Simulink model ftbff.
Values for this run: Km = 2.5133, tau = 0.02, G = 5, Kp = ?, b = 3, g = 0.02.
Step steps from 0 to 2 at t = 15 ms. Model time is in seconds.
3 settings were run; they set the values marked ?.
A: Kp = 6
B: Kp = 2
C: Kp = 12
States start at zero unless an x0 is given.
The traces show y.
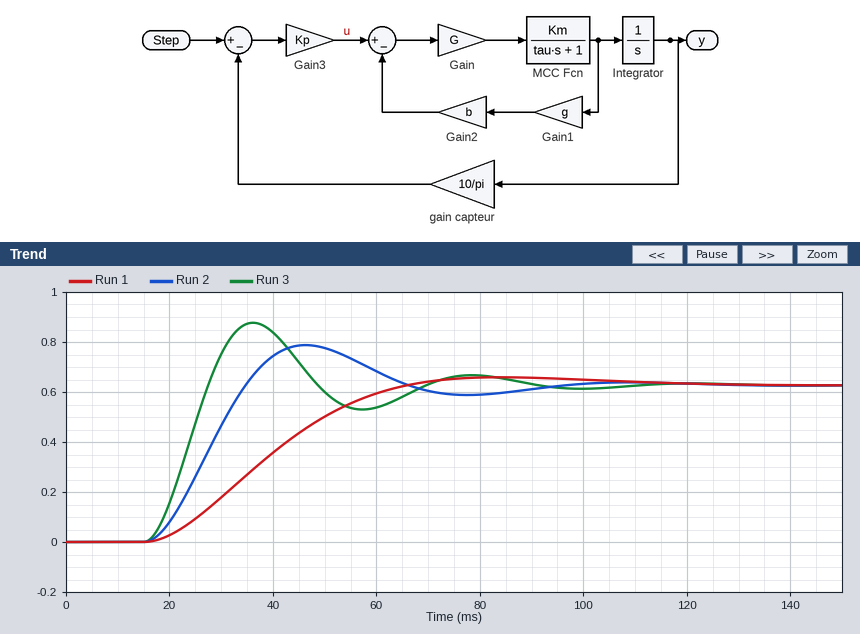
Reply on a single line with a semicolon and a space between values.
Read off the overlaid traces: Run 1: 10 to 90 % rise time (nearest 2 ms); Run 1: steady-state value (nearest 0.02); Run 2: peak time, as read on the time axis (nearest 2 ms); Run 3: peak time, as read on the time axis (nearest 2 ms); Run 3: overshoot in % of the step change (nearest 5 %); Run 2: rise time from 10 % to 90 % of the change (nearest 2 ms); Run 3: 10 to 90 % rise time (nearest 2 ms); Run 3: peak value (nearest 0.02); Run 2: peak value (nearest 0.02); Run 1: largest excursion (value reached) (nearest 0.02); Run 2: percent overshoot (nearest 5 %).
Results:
34 ms; 0.62; 46 ms; 36 ms; 40 %; 14 ms; 8 ms; 0.88; 0.78; 0.66; 25 %
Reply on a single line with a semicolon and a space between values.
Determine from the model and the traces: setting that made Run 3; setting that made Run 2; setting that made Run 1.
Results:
C; A; B
